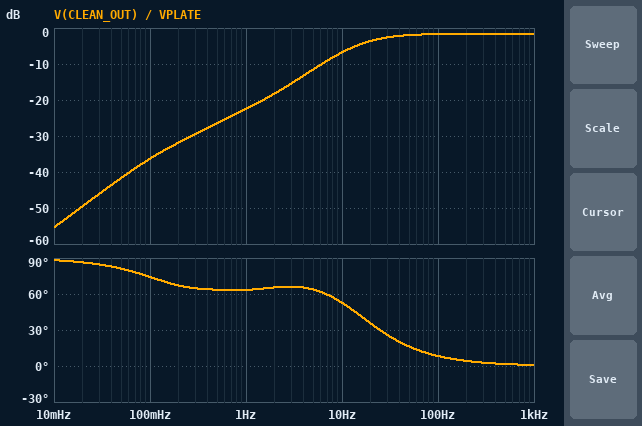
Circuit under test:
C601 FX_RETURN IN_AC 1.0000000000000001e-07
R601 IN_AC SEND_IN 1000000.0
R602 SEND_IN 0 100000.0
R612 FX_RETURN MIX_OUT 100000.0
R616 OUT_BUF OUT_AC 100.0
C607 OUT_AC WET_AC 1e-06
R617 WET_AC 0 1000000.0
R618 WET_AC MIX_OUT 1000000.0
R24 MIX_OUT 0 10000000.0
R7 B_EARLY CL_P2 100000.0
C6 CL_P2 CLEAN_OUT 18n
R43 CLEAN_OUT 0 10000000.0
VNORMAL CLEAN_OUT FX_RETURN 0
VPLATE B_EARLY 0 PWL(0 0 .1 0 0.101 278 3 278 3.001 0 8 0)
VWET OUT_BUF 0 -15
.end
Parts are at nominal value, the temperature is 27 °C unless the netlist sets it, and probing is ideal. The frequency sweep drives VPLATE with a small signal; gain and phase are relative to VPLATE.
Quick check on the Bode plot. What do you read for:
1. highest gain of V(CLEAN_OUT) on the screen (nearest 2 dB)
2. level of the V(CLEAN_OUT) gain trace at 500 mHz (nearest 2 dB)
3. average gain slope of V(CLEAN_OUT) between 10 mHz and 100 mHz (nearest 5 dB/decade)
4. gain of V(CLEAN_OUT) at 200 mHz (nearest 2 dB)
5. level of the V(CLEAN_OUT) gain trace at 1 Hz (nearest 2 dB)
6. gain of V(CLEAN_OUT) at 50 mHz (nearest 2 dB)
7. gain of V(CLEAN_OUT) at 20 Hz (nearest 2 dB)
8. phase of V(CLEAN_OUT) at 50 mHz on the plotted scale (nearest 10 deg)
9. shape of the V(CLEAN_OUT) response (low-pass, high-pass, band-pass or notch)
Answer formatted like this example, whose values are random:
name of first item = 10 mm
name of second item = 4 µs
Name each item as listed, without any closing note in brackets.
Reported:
highest gain of V(CLEAN_OUT) on the screen = -2 dB
level of the V(CLEAN_OUT) gain trace at 500 mHz = -26 dB
average gain slope of V(CLEAN_OUT) between 10 mHz and 100 mHz = 20 dB/decade
gain of V(CLEAN_OUT) at 200 mHz = -32 dB
level of the V(CLEAN_OUT) gain trace at 1 Hz = -22 dB
gain of V(CLEAN_OUT) at 50 mHz = -42 dB
gain of V(CLEAN_OUT) at 20 Hz = -4 dB
phase of V(CLEAN_OUT) at 50 mHz on the plotted scale = 80 deg
shape of the V(CLEAN_OUT) response = high-pass
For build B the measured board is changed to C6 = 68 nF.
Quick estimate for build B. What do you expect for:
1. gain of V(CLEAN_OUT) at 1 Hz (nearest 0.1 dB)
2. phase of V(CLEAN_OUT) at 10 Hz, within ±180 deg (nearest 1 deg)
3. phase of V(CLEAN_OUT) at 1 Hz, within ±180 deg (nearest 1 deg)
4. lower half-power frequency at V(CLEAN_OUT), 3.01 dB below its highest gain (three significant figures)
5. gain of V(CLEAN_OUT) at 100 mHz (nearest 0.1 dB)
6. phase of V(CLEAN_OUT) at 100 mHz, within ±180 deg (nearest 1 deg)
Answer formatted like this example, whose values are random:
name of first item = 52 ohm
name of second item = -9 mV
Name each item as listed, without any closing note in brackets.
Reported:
gain of V(CLEAN_OUT) at 1 Hz = -11.9 dB
phase of V(CLEAN_OUT) at 10 Hz, within ±180 deg = 20 deg
phase of V(CLEAN_OUT) at 1 Hz, within ±180 deg = 52 deg
lower half-power frequency at V(CLEAN_OUT), 3.01 dB below its highest gain = 4.26 Hz
gain of V(CLEAN_OUT) at 100 mHz = -24.9 dB
phase of V(CLEAN_OUT) at 100 mHz, within ±180 deg = 72 deg
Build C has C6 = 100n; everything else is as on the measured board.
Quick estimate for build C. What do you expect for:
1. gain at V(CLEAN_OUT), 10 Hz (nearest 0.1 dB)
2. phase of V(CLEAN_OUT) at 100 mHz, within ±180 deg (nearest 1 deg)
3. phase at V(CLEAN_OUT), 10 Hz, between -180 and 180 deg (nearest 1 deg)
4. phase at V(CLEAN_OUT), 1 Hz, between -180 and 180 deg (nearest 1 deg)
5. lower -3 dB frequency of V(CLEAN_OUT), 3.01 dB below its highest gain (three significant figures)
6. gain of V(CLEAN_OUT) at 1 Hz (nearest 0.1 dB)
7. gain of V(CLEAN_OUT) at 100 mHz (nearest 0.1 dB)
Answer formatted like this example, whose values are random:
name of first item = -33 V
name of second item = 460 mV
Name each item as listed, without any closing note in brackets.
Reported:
gain at V(CLEAN_OUT), 10 Hz = -2.0 dB
phase of V(CLEAN_OUT) at 100 mHz, within ±180 deg = 70 deg
phase at V(CLEAN_OUT), 10 Hz, between -180 and 180 deg = 14 deg
phase at V(CLEAN_OUT), 1 Hz, between -180 and 180 deg = 46 deg
lower -3 dB frequency of V(CLEAN_OUT), 3.01 dB below its highest gain = 2.91 Hz
gain of V(CLEAN_OUT) at 1 Hz = -9.2 dB
gain of V(CLEAN_OUT) at 100 mHz = -21.6 dB
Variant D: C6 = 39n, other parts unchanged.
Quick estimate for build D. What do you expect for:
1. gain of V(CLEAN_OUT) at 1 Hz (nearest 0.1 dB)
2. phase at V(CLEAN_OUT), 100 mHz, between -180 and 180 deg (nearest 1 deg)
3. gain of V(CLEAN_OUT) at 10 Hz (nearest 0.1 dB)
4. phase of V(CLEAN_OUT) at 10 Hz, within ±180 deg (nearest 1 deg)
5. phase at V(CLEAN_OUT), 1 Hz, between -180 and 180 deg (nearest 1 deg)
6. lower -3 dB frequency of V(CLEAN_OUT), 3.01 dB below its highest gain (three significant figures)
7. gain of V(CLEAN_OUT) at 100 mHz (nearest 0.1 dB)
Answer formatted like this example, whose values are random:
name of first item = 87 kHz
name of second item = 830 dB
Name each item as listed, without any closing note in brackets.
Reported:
gain of V(CLEAN_OUT) at 1 Hz = -16.1 dB
phase at V(CLEAN_OUT), 100 mHz, between -180 and 180 deg = 73 deg
gain of V(CLEAN_OUT) at 10 Hz = -3.4 dB
phase of V(CLEAN_OUT) at 10 Hz, within ±180 deg = 32 deg
phase at V(CLEAN_OUT), 1 Hz, between -180 and 180 deg = 58 deg
lower -3 dB frequency of V(CLEAN_OUT), 3.01 dB below its highest gain = 7.26 Hz
gain of V(CLEAN_OUT) at 100 mHz = -29.6 dB
